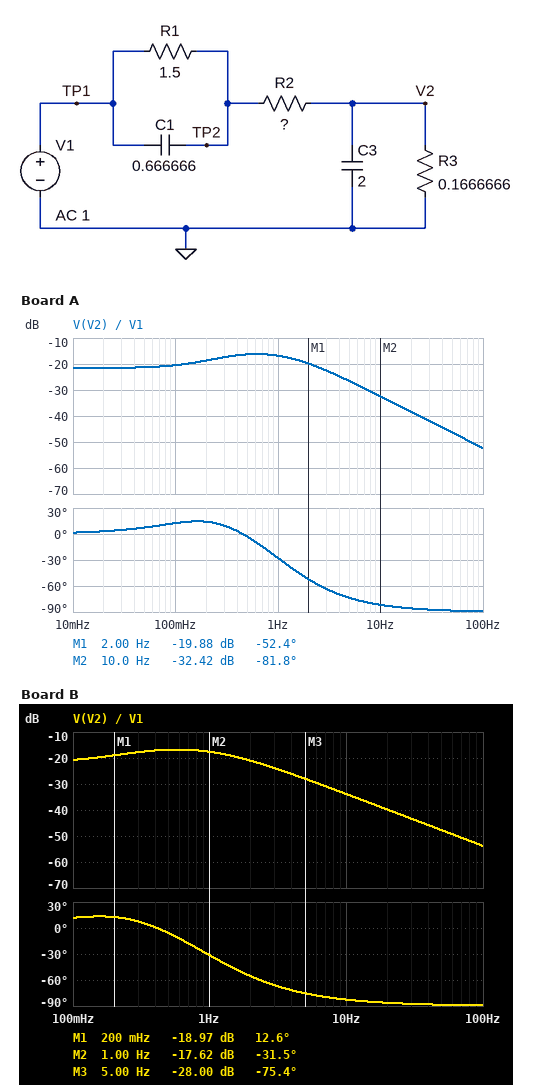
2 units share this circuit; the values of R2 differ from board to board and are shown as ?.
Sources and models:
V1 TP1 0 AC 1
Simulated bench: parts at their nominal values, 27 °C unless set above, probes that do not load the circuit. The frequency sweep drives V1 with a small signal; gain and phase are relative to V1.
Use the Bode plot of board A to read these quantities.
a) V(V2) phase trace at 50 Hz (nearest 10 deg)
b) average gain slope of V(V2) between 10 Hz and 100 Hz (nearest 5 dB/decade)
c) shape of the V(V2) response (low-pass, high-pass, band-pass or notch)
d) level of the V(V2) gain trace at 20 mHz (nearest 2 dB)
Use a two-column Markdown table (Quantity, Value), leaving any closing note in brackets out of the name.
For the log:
| Quantity | Value |
|---|---|
| V(V2) phase trace at 50 Hz | -90 deg |
| average gain slope of V(V2) between 10 Hz and 100 Hz | -20 dB/decade |
| shape of the V(V2) response | low-pass |
| level of the V(V2) gain trace at 20 mHz | -22 dB |
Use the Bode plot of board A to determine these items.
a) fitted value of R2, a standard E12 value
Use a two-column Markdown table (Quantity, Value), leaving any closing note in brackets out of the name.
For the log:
| Quantity | Value |
|---|---|
| fitted value of R2, a standard E12 value | 0.33 Ω |
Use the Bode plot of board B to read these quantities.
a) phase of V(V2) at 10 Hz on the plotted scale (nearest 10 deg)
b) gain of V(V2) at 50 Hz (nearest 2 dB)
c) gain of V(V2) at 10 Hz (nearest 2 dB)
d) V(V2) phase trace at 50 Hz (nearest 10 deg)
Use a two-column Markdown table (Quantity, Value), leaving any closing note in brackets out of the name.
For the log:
| Quantity | Value |
|---|---|
| phase of V(V2) at 10 Hz on the plotted scale | -80 deg |
| gain of V(V2) at 50 Hz | -48 dB |
| gain of V(V2) at 10 Hz | -34 dB |
| V(V2) phase trace at 50 Hz | -90 deg |
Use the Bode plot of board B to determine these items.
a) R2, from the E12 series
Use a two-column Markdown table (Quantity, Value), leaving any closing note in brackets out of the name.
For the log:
| Quantity | Value |
|---|---|
| R2, from the E12 series | 0.39 Ω |
